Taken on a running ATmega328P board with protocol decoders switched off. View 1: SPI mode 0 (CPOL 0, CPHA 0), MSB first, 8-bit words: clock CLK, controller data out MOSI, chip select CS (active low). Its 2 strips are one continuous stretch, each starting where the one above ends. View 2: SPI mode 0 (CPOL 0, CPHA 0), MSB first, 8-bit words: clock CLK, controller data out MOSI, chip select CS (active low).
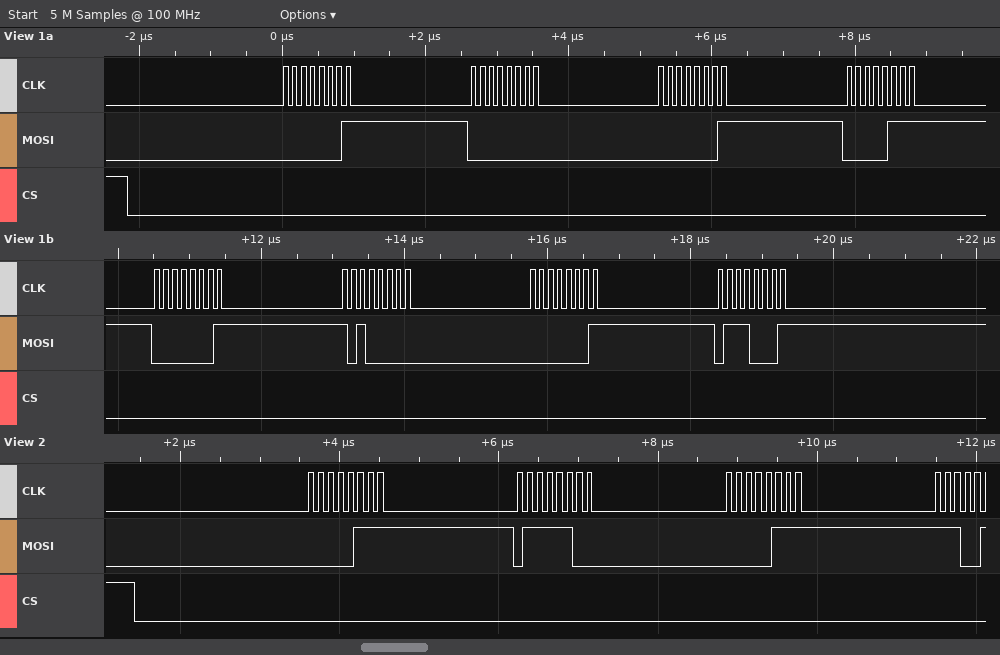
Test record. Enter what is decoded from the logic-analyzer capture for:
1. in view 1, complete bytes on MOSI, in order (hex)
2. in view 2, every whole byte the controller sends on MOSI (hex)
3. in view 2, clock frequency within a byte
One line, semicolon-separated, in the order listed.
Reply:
01 00 01 07 01 A0 01 71; 0x07 0x7C 0x07; 8 MHz
